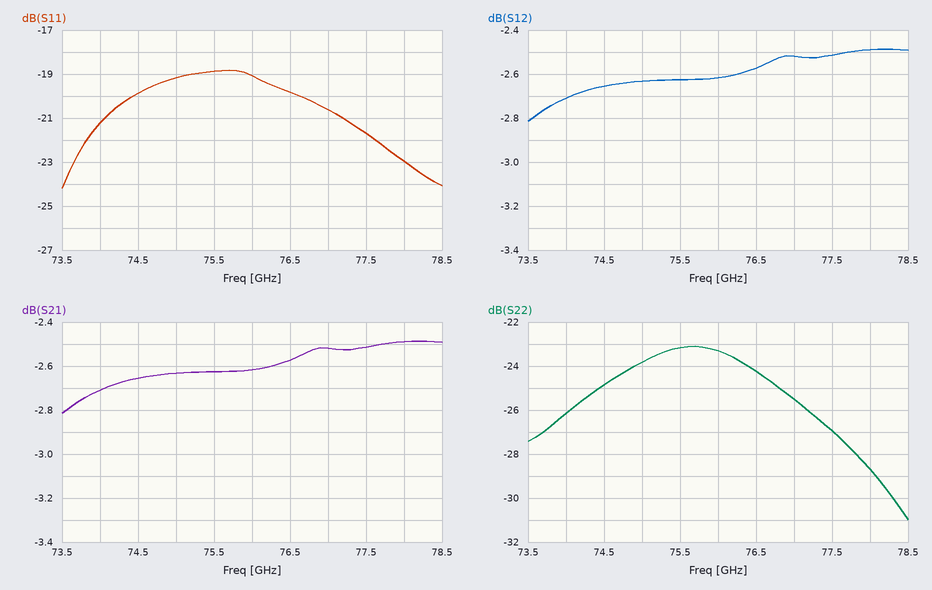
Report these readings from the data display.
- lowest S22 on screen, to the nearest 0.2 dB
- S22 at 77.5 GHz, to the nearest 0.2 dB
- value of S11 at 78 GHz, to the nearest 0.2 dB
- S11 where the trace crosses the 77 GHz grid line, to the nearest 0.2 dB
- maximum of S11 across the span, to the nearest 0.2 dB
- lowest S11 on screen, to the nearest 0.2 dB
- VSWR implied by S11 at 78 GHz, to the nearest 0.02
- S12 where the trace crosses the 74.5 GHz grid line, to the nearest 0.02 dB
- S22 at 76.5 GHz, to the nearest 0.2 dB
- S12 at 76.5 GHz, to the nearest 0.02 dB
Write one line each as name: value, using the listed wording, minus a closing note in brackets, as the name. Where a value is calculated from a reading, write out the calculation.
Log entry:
lowest S22 on screen, to the nearest 0.2 dB: -31.0 dB
S22 at 77.5 GHz, to the nearest 0.2 dB: -27.0 dB
value of S11 at 78 GHz, to the nearest 0.2 dB: -23.0 dB
S11 where the trace crosses the 77 GHz grid line, to the nearest 0.2 dB: -20.6 dB
maximum of S11 across the span, to the nearest 0.2 dB: -18.8 dB
lowest S11 on screen, to the nearest 0.2 dB: -24.2 dB
VSWR implied by S11 at 78 GHz, to the nearest 0.02: |Γ| = 10^(-23/20) = 0.0708; VSWR = (1 + 0.0708)/(1 − 0.0708) ≈ 1.15, so 1.16 to the nearest 0.02
S12 where the trace crosses the 74.5 GHz grid line, to the nearest 0.02 dB: -2.66 dB
S22 at 76.5 GHz, to the nearest 0.2 dB: -24.2 dB
S12 at 76.5 GHz, to the nearest 0.02 dB: -2.58 dB
